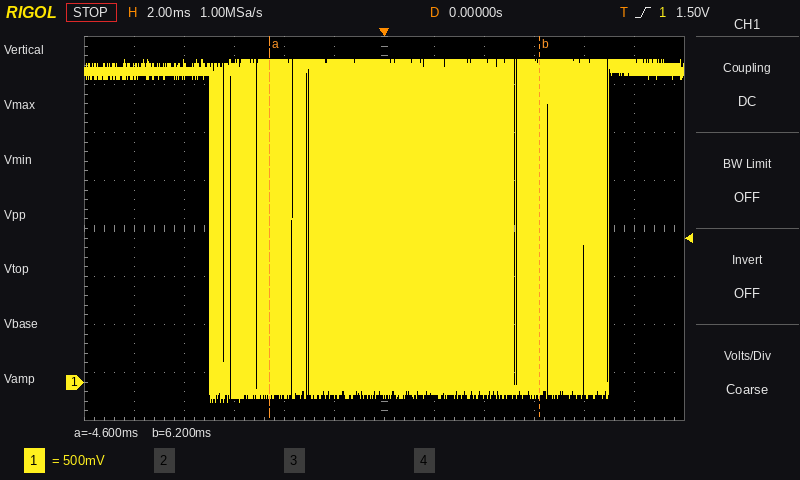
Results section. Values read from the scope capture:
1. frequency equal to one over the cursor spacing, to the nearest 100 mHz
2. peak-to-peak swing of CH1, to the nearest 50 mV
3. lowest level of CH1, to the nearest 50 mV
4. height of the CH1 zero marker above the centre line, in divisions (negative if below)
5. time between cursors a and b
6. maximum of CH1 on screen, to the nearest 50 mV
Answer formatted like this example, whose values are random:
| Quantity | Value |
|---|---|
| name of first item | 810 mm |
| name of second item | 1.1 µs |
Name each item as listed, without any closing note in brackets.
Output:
| Quantity | Value |
|---|---|
| frequency equal to one over the cursor spacing, to the nearest 100 mHz | 92.6 Hz |
| peak-to-peak swing of CH1, to the nearest 50 mV | 3.55 V |
| lowest level of CH1, to the nearest 50 mV | -200 mV |
| height of the CH1 zero marker above the centre line, in divisions | -3.2 div |
| time between cursors a and b | 10.8 ms |
| maximum of CH1 on screen, to the nearest 50 mV | 3.35 V |
